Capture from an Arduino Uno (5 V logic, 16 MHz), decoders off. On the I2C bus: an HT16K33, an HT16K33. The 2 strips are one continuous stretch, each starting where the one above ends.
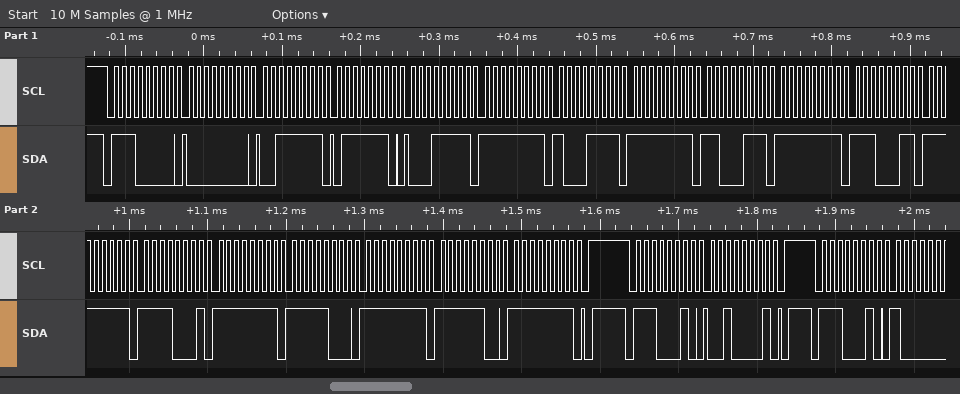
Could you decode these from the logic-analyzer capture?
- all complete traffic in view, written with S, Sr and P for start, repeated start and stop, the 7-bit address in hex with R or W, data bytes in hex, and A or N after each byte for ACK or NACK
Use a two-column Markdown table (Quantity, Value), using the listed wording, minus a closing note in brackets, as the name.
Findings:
| Quantity | Value |
|---|---|
| all complete traffic in view, written with S, Sr and P for start, repeated start and stop, the 7-bit address in hex with R or W, data bytes in hex, and A or N after each byte for ACK or NACK | S 70W A 00 A 3F A 7E A 1F A FF A 8F A FF A C7 A FF A E3 A FF A F1 A FF A F8 A FF A FC A FF A P S 71W A 21 A P S 71W A |
